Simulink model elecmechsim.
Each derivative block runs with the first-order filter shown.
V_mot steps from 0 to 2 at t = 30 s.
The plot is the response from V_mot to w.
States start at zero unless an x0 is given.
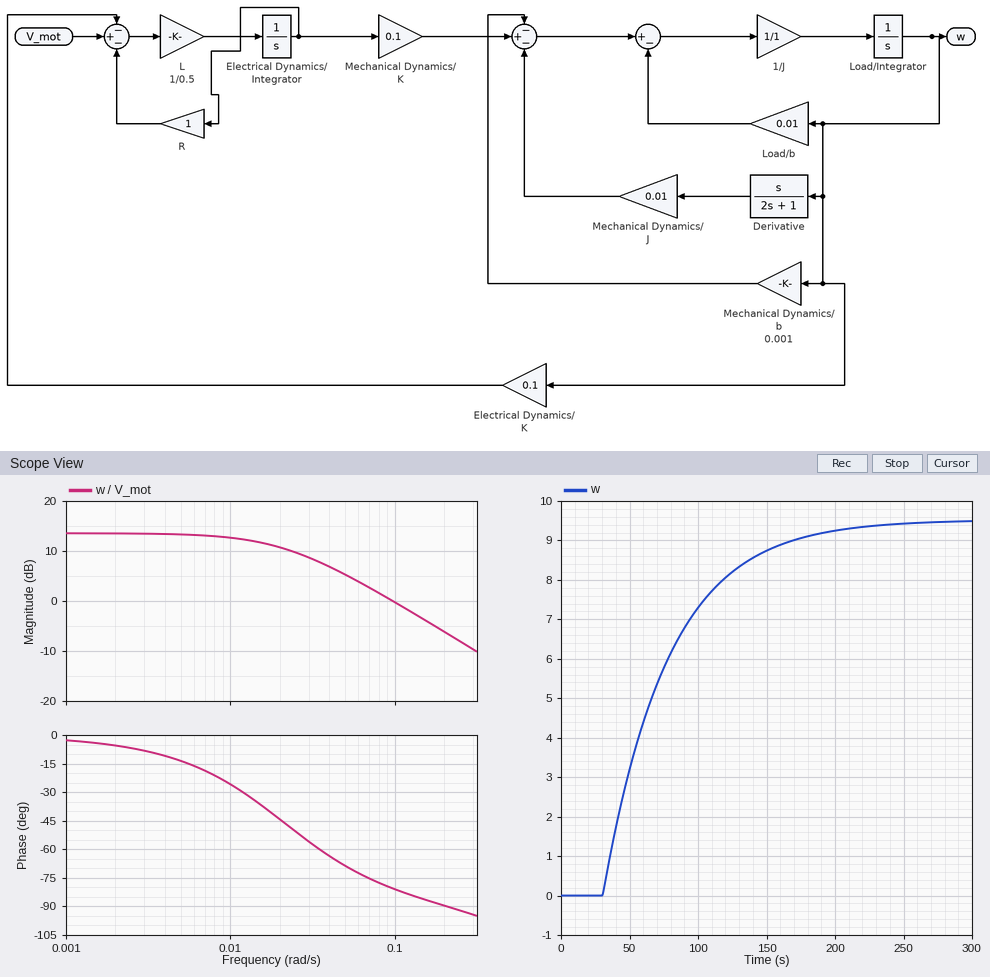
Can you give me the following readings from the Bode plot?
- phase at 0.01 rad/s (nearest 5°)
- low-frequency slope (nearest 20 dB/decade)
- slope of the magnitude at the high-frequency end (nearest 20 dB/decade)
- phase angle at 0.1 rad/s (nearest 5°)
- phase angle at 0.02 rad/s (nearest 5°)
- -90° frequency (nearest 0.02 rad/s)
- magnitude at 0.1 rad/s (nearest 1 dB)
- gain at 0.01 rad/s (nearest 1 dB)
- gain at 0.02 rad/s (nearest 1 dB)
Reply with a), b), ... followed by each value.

a) -25°
b) 0 dB/decade
c) -20 dB/decade
d) -80°
e) -45°
f) 0.20 rad/s
g) 0 dB
h) 13 dB
i) 11 dB
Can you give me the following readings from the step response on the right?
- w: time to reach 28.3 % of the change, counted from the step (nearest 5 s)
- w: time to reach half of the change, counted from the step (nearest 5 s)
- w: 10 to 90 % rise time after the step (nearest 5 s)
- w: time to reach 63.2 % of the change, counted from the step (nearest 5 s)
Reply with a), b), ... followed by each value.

a) 15 s
b) 35 s
c) 105 s
d) 50 s
